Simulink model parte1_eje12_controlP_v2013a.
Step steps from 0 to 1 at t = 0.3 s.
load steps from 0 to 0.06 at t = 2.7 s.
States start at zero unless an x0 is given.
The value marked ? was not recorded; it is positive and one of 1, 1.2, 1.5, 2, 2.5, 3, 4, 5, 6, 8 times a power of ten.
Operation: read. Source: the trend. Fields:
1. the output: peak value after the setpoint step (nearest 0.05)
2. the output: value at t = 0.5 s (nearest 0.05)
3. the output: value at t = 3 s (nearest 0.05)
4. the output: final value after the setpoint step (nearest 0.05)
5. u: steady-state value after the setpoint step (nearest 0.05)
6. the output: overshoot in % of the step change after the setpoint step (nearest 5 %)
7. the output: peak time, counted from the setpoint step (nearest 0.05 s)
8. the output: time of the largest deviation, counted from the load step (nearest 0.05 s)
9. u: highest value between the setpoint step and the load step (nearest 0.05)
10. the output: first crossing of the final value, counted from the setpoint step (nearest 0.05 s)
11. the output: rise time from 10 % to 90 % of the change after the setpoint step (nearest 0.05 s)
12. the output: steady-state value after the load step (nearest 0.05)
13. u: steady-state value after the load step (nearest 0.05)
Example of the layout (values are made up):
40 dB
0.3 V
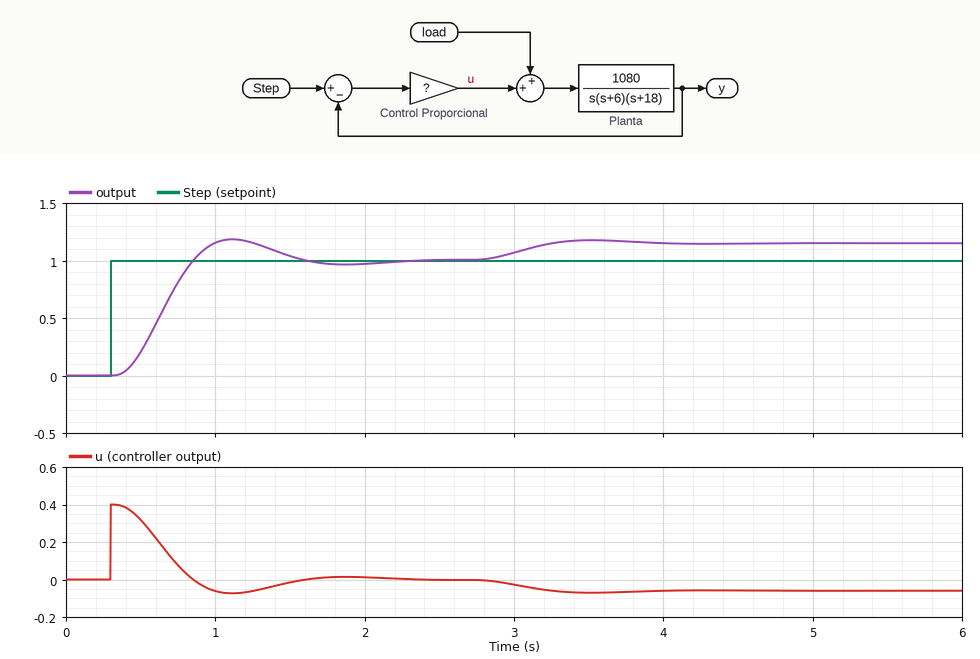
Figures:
1.20
0.20
1.05
1.00
0.00
20 %
0.80 s
0.80 s
0.40
0.55 s
0.35 s
1.15
-0.05
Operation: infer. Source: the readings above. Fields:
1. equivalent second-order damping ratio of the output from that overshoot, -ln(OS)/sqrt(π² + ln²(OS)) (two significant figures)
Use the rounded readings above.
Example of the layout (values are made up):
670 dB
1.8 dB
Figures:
0.46
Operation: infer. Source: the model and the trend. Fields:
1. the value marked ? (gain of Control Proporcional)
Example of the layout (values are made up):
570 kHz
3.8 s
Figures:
0.4
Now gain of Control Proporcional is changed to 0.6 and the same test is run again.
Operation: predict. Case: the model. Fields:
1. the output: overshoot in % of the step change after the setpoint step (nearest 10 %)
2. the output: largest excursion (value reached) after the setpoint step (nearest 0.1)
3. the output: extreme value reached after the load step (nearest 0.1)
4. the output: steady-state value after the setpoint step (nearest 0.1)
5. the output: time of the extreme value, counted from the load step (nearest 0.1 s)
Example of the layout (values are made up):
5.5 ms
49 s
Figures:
30 %
1.3
1.1
1.0
0.6 s
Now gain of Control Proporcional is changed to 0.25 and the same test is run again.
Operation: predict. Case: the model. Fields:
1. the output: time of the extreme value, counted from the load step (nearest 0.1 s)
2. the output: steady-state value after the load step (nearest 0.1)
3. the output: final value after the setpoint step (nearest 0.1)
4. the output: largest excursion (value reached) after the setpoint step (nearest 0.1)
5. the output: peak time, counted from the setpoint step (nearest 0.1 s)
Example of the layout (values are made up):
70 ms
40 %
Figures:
1.2 s
1.2
1.0
1.1
1.2 s
